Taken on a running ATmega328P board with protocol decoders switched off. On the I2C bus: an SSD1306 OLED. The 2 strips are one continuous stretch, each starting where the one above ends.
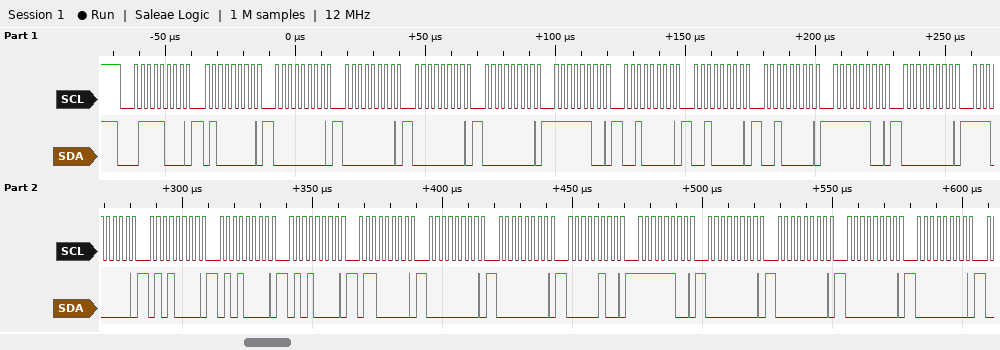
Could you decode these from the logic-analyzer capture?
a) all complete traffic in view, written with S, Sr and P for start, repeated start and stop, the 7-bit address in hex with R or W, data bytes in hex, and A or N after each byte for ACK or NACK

S 3CW A 40 A 00 A 00 A 00 A 00 A FC A 20 A 20 A 20 A FC A 00 A E0 A 50 A 50 A 50 A 60 A 00 A 00 A 04 A FC A 00 A 00 A 00 A 00 A
